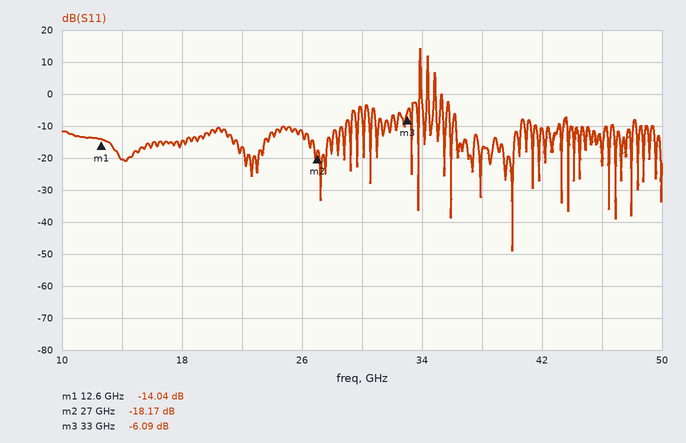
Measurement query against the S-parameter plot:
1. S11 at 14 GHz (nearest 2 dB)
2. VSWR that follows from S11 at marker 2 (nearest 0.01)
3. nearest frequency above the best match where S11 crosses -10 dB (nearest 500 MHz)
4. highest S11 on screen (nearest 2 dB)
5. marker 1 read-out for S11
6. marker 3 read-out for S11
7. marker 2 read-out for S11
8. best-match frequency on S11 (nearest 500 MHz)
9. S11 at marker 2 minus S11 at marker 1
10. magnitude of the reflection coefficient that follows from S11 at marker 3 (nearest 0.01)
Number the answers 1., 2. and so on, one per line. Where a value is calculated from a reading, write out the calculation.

1. -20 dB
2. (1 + 0.1235)/(1 − 0.1235) ≈ 1.28
3. 40.5 GHz
4. 14 dB
5. -14.04 dB
6. -6.09 dB
7. -18.17 dB
8. 40.0 GHz
9. -18.17 − (-14.04) = -4.13 dB
10. 10^(-6.09/20) ≈ 0.50
